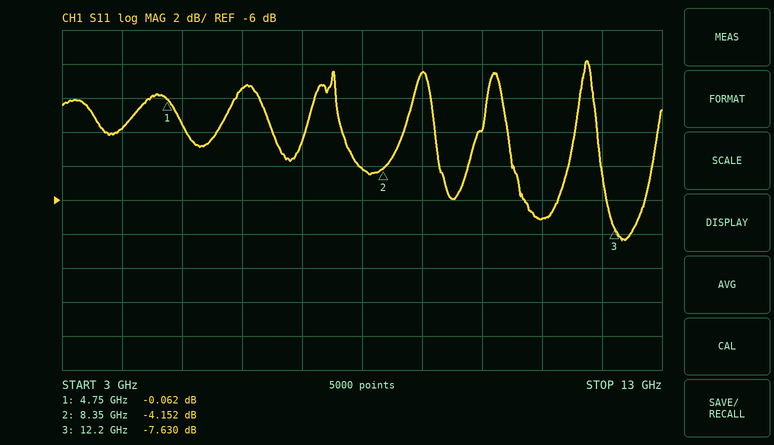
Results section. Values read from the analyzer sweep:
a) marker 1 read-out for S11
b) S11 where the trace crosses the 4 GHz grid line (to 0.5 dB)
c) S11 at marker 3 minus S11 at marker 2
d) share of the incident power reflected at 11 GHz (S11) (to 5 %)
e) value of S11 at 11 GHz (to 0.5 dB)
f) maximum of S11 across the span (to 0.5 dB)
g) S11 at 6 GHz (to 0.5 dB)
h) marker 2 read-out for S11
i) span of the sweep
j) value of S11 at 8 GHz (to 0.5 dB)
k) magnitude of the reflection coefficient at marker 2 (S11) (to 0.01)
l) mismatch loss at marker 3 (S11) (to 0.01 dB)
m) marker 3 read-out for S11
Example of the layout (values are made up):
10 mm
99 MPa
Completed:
-0.062 dB
-2.0 dB
-3.478 dB
20 %
-7.0 dB
2.0 dB
0.5 dB
-4.152 dB
10 GHz
-4.0 dB
0.62
0.82 dB
-7.630 dB
